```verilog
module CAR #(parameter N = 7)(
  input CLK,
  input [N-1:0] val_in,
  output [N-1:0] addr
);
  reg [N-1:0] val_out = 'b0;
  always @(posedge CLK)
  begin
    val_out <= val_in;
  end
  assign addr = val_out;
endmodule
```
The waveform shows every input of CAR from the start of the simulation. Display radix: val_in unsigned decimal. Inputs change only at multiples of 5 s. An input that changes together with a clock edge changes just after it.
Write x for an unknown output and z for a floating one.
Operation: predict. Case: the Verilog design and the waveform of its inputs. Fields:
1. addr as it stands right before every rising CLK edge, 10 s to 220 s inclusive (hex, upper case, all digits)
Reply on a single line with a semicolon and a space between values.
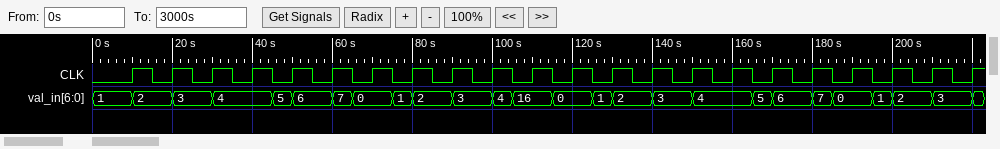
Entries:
00, 01, 02, 03, 04, 05, 06, 00, 01, 02, 03, 10, 00, 01, 02, 03, 04, 05, 06, 00, 01, 02
